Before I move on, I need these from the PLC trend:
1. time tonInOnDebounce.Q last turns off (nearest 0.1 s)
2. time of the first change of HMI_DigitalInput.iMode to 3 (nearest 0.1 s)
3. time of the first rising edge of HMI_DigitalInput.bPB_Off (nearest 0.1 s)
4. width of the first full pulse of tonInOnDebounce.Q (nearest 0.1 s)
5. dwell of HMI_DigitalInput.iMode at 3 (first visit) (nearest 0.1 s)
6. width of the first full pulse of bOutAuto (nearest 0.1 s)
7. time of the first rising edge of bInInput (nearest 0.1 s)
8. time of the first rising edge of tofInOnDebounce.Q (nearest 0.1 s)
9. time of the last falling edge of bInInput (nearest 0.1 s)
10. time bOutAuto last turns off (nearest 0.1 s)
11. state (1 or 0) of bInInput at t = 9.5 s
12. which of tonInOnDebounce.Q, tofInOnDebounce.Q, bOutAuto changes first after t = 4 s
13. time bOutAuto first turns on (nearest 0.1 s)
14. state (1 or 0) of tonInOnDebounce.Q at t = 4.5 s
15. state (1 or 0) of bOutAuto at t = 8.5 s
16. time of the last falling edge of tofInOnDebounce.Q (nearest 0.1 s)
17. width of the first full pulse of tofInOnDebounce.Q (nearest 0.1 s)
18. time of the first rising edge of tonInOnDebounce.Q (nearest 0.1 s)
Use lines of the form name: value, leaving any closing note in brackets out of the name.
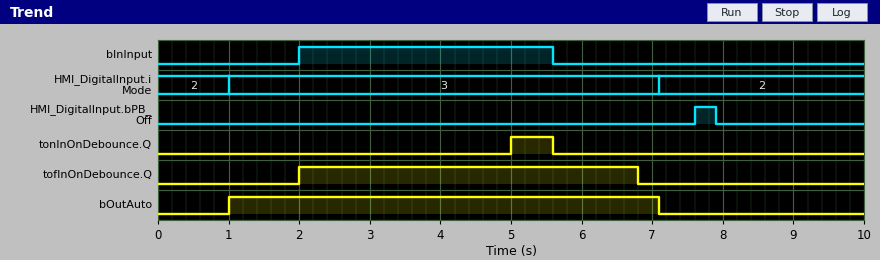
time tonInOnDebounce.Q last turns off: 5.6 s
time of the first change of HMI_DigitalInput.iMode to 3: 1.0 s
time of the first rising edge of HMI_DigitalInput.bPB_Off: 7.6 s
width of the first full pulse of tonInOnDebounce.Q: 0.6 s
dwell of HMI_DigitalInput.iMode at 3 (first visit): 6.1 s
width of the first full pulse of bOutAuto: 6.1 s
time of the first rising edge of bInInput: 2.0 s
time of the first rising edge of tofInOnDebounce.Q: 2.0 s
time of the last falling edge of bInInput: 5.6 s
time bOutAuto last turns off: 7.1 s
state (1 or 0) of bInInput at t = 9.5 s: 0
which of tonInOnDebounce.Q, tofInOnDebounce.Q, bOutAuto changes first after t = 4 s: tonInOnDebounce.Q
time bOutAuto first turns on: 1.0 s
state (1 or 0) of tonInOnDebounce.Q at t = 4.5 s: 0
state (1 or 0) of bOutAuto at t = 8.5 s: 0
time of the last falling edge of tofInOnDebounce.Q: 6.8 s
width of the first full pulse of tofInOnDebounce.Q: 4.8 s
time of the first rising edge of tonInOnDebounce.Q: 5.0 s
